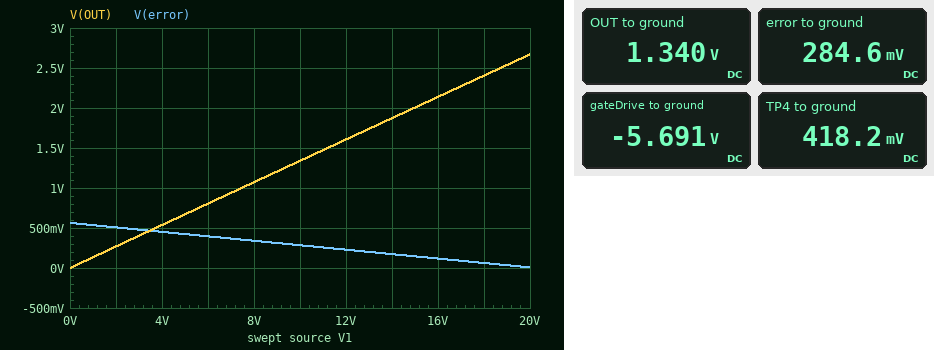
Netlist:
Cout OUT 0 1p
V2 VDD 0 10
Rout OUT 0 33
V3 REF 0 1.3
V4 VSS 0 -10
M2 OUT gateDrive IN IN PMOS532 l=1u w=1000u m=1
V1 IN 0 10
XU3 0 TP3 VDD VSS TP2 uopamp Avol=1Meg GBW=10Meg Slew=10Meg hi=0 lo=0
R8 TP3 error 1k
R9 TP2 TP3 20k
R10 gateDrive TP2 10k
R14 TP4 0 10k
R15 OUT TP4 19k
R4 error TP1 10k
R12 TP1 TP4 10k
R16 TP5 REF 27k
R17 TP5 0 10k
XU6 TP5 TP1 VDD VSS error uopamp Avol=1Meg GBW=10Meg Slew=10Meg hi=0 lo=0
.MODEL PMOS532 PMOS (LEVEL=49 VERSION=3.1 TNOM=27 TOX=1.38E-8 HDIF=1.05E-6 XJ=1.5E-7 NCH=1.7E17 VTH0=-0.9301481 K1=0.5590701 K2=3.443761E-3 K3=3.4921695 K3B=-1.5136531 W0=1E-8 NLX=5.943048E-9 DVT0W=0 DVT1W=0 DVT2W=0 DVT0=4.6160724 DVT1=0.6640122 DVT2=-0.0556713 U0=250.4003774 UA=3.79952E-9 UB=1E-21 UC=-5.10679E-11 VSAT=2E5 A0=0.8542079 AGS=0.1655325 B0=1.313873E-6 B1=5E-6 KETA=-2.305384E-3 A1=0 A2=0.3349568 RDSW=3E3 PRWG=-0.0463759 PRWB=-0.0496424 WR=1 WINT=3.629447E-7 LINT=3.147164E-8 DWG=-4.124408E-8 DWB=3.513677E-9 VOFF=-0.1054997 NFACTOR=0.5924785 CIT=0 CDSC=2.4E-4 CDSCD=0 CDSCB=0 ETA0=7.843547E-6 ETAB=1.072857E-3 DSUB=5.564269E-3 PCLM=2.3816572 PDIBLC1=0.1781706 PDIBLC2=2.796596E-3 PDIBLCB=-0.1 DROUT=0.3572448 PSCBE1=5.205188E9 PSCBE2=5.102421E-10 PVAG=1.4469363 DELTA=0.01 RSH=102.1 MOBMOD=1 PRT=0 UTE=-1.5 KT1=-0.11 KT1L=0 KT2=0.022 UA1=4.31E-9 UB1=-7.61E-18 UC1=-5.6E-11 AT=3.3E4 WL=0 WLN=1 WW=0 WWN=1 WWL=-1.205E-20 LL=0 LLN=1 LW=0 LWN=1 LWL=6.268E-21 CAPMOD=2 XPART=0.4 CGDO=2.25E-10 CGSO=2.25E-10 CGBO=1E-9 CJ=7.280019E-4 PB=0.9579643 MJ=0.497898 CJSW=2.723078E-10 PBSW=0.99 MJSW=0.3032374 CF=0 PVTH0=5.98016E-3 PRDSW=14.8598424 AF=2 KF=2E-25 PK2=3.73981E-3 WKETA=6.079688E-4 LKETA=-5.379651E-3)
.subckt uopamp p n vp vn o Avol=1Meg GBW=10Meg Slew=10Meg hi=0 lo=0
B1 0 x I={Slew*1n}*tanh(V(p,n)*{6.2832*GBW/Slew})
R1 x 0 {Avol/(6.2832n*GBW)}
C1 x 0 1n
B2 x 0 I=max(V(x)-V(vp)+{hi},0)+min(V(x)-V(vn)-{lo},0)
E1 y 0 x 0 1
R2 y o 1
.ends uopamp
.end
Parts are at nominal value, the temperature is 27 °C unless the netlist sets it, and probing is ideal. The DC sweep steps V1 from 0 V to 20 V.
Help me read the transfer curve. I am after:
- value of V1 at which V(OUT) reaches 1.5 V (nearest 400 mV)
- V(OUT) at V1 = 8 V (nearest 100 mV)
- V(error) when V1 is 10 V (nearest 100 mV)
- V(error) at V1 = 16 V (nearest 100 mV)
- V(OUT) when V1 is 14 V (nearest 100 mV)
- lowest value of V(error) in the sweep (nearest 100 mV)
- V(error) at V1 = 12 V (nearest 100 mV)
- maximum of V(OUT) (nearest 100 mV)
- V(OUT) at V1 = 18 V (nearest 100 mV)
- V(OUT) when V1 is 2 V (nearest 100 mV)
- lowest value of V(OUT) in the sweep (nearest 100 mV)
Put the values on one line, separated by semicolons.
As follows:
11.2 V; 1.1 V; 300 mV; 100 mV; 1.9 V; 0 V; 200 mV; 2.7 V; 2.4 V; 300 mV; 0 V
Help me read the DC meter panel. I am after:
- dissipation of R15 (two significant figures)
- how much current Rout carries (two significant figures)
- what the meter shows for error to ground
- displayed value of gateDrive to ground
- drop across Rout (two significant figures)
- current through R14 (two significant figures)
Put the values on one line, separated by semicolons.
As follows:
45 µW; 41 mA; 284.6 mV; -5.691 V; 1.3 V; 42 µA
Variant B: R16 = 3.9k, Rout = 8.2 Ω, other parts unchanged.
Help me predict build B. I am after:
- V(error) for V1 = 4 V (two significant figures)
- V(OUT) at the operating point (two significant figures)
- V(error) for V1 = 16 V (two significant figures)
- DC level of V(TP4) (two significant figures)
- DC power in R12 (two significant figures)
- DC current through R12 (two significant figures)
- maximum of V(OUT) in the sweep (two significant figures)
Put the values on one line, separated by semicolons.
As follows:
1.5 V; 370 mV; 1.4 V; 450 mV; 24 µW; 49 µA; 750 mV
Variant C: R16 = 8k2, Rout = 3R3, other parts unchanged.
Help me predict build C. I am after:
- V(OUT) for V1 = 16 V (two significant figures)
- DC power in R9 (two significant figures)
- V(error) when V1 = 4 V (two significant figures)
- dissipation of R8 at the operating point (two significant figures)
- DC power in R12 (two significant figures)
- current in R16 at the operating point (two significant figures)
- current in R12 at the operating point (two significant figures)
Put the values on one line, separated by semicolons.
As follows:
250 mV; 5.6 mW; 1.1 V; 280 µW; 16 µW; 71 µA; 40 µA
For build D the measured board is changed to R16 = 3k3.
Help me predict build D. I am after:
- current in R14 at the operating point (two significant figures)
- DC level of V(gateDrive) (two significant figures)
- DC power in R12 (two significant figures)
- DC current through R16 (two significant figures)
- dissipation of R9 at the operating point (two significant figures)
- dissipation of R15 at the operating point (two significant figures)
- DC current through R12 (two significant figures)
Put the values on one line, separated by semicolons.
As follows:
67 µA; -10 V; 9.6 µW; 98 µA; 5.8 mW; 24 µW; 31 µA
